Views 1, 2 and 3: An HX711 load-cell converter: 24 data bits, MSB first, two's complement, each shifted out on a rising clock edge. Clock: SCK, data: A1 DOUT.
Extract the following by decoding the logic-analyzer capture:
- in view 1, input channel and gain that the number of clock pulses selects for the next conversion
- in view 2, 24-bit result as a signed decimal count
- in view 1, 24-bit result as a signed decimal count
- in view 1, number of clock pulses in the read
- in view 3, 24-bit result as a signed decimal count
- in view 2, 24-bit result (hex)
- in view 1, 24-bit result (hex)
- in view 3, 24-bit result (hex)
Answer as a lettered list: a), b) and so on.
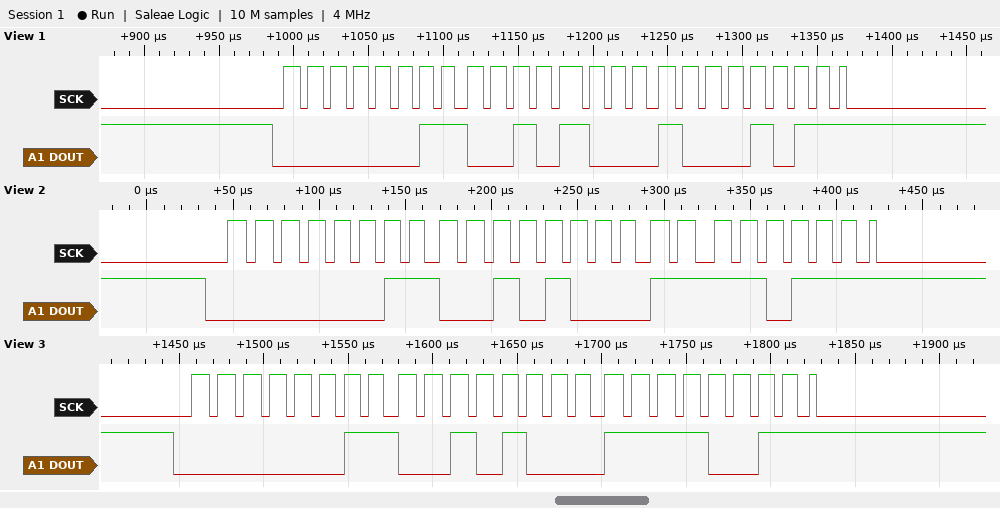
a) channel A, gain 128
b) 207095
c) 206987
d) 25
e) 207091
f) 0x0328F7
g) 0x03288B
h) 0x0328F3
